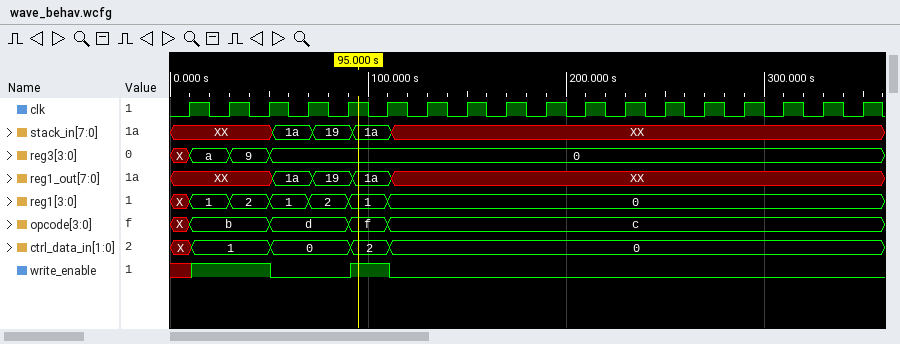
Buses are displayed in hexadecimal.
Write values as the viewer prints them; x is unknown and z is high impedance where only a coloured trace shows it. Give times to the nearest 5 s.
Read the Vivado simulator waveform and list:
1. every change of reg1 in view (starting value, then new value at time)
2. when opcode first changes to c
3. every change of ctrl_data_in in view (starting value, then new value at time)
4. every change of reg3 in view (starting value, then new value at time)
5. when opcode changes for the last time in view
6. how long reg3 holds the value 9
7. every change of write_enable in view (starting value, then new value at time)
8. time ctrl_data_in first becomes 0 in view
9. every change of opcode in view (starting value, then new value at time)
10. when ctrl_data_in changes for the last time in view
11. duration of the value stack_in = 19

X, 1 at 10 s, 2 at 30 s, 1 at 50 s, 2 at 70 s, 1 at 90 s, 0 at 110 s
110 s
X, 1 at 10 s, 0 at 50 s, 2 at 90 s, 0 at 110 s
X, a at 10 s, 9 at 30 s, 0 at 50 s
110 s
20 s
x, 1 at 10 s, 0 at 50 s, 1 at 90 s, 0 at 110 s
50 s
X, b at 10 s, d at 50 s, f at 90 s, c at 110 s
110 s
20 s
